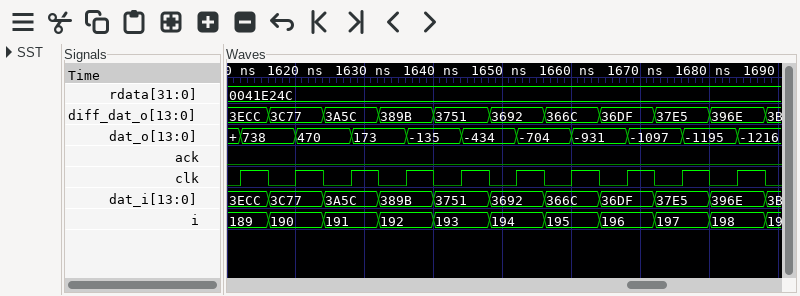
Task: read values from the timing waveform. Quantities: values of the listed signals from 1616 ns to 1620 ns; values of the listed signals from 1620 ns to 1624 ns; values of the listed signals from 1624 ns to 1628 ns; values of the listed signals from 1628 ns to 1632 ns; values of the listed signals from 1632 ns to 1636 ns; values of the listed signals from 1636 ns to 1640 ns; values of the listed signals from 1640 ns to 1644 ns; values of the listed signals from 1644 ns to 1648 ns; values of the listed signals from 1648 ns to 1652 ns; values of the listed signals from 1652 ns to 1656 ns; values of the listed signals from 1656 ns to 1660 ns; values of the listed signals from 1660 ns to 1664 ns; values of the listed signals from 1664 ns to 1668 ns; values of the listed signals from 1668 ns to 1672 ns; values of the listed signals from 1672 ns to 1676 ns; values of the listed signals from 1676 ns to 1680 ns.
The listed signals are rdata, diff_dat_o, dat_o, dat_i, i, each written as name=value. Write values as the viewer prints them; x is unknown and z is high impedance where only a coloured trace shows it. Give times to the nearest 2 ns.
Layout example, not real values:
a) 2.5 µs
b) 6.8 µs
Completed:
a) rdata=0041E24C, diff_dat_o=3C77, dat_o=738, dat_i=3C77, i=190
b) rdata=0041E24C, diff_dat_o=3C77, dat_o=470, dat_i=3C77, i=190
c) rdata=0041E24C, diff_dat_o=3A5C, dat_o=470, dat_i=3A5C, i=191
d) rdata=0041E24C, diff_dat_o=3A5C, dat_o=173, dat_i=3A5C, i=191
e) rdata=0041E24C, diff_dat_o=389B, dat_o=173, dat_i=389B, i=192
f) rdata=0041E24C, diff_dat_o=389B, dat_o=-135, dat_i=389B, i=192
g) rdata=0041E24C, diff_dat_o=3751, dat_o=-135, dat_i=3751, i=193
h) rdata=0041E24C, diff_dat_o=3751, dat_o=-434, dat_i=3751, i=193
i) rdata=0041E24C, diff_dat_o=3692, dat_o=-434, dat_i=3692, i=194
j) rdata=0041E24C, diff_dat_o=3692, dat_o=-704, dat_i=3692, i=194
k) rdata=0041E24C, diff_dat_o=366C, dat_o=-704, dat_i=366C, i=195
l) rdata=0041E24C, diff_dat_o=366C, dat_o=-931, dat_i=366C, i=195
m) rdata=0041E24C, diff_dat_o=36DF, dat_o=-931, dat_i=36DF, i=196
n) rdata=0041E24C, diff_dat_o=36DF, dat_o=-1097, dat_i=36DF, i=196
o) rdata=0041E24C, diff_dat_o=37E5, dat_o=-1097, dat_i=37E5, i=197
p) rdata=0041E24C, diff_dat_o=37E5, dat_o=-1195, dat_i=37E5, i=197
